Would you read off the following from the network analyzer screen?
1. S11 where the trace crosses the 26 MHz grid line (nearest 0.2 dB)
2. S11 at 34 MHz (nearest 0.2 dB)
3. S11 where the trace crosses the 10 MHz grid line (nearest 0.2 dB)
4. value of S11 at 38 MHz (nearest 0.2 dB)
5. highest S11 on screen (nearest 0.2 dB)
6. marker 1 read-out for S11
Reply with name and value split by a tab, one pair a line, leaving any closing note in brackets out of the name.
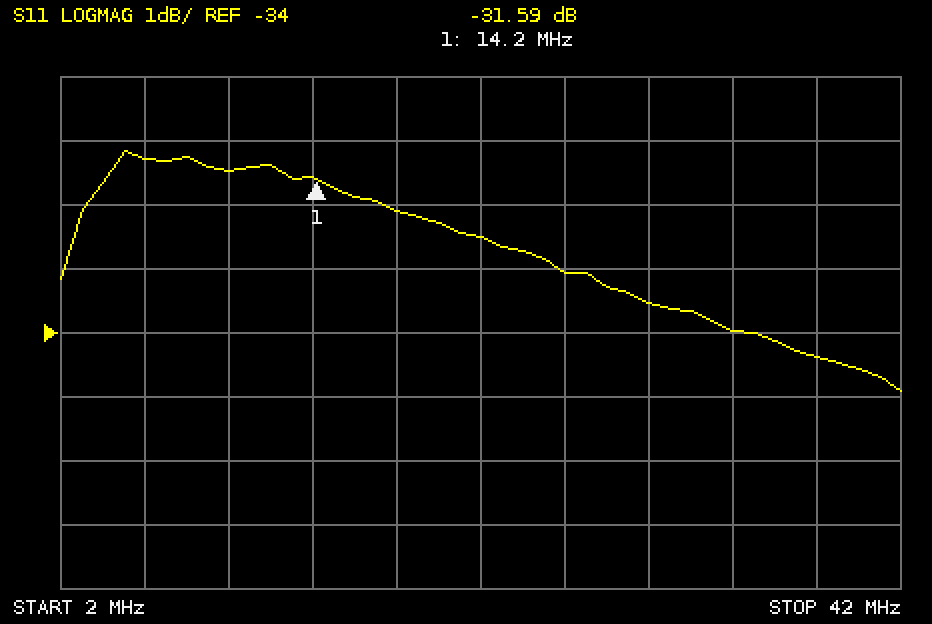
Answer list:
S11 where the trace crosses the 26 MHz grid line	-33.0 dB
S11 at 34 MHz	-34.0 dB
S11 where the trace crosses the 10 MHz grid line	-31.4 dB
value of S11 at 38 MHz	-34.4 dB
highest S11 on screen	-31.2 dB
marker 1 read-out for S11	-31.59 dB
